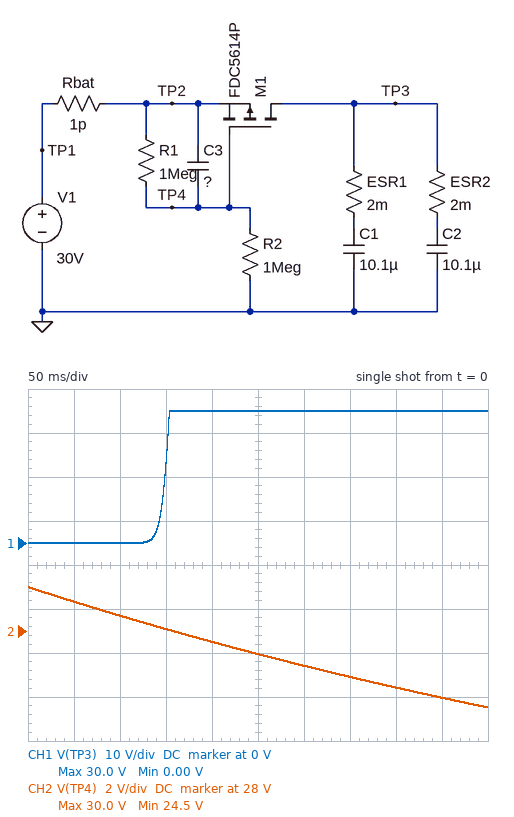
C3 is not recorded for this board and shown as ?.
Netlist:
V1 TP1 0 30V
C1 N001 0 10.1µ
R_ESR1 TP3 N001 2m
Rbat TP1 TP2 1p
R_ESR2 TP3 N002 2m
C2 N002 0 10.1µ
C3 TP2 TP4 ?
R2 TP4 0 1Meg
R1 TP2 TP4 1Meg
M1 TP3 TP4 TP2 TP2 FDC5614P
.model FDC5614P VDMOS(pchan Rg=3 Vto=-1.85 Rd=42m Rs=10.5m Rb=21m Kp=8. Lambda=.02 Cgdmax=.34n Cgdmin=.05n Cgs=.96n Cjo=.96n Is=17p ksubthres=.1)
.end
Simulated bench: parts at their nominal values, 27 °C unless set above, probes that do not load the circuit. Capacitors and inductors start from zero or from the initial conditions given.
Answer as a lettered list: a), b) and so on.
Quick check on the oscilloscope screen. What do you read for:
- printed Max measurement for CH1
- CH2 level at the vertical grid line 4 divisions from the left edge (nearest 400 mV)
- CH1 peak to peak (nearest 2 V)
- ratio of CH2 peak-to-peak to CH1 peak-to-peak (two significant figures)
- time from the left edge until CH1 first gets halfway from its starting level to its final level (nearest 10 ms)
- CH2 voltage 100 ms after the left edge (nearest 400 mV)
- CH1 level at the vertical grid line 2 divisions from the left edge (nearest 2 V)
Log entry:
a) 30.0 V
b) 27.6 V
c) 30 V
d) 0.18
e) 150 ms
f) 28.8 V
g) 0 V
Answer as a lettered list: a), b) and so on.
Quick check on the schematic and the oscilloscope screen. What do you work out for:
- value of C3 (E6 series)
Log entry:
a) 2.2 µF
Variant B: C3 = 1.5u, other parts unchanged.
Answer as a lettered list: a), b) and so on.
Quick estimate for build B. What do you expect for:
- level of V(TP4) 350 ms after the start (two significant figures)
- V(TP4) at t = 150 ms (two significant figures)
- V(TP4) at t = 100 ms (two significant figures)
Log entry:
a) 24 V
b) 27 V
c) 28 V
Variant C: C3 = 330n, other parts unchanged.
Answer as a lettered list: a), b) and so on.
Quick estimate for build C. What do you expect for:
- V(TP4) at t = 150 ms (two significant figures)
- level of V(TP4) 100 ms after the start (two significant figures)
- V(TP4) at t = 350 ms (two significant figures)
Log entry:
a) 21 V
b) 23 V
c) 17 V
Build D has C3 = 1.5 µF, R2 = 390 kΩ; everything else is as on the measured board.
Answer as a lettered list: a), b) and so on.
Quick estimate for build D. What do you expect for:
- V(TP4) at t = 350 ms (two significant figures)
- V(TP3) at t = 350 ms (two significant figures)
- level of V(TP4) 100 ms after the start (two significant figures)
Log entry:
a) 18 V
b) 30 V
c) 25 V
